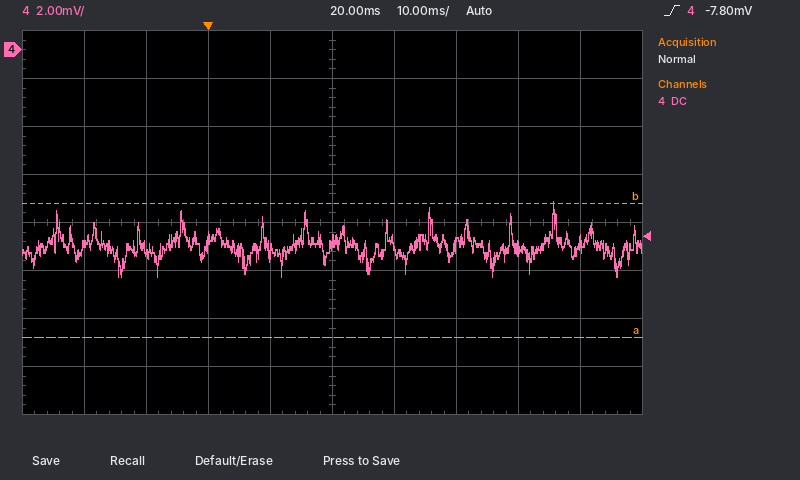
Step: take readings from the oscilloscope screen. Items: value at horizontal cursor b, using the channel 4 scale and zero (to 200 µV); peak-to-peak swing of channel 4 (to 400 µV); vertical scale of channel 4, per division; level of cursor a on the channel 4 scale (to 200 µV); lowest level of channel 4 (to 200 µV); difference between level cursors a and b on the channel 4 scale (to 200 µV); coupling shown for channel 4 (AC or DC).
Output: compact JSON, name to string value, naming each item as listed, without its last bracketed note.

{"value at horizontal cursor b, using the channel 4 scale and zero": "-6.4 mV", "peak-to-peak swing of channel 4": "3.2 mV", "vertical scale of channel 4, per division": "2 mV", "level of cursor a on the channel 4 scale": "-12.0 mV", "lowest level of channel 4": "-9.4 mV", "difference between level cursors a and b on the channel 4 scale": "5.6 mV", "coupling shown for channel 4": "DC"}
